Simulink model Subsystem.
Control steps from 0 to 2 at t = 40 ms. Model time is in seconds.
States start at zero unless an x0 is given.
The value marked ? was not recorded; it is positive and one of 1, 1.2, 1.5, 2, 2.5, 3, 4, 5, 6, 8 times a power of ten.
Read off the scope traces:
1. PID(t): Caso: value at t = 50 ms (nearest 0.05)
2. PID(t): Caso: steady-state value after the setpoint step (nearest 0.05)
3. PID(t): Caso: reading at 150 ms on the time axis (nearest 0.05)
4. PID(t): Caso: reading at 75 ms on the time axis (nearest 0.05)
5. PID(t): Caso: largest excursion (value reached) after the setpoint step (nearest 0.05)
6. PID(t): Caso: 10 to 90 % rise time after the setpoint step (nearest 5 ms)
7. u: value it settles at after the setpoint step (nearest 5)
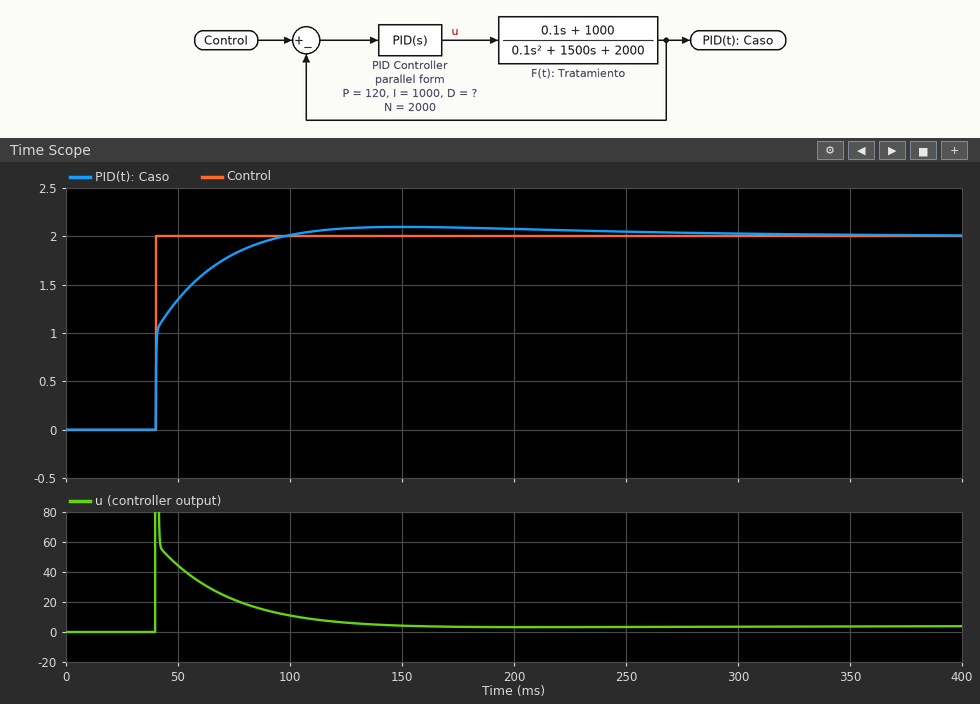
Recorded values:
1.35
2.00
2.10
1.80
2.10
35 ms
5
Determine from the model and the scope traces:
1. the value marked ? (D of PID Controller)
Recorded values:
1.5
